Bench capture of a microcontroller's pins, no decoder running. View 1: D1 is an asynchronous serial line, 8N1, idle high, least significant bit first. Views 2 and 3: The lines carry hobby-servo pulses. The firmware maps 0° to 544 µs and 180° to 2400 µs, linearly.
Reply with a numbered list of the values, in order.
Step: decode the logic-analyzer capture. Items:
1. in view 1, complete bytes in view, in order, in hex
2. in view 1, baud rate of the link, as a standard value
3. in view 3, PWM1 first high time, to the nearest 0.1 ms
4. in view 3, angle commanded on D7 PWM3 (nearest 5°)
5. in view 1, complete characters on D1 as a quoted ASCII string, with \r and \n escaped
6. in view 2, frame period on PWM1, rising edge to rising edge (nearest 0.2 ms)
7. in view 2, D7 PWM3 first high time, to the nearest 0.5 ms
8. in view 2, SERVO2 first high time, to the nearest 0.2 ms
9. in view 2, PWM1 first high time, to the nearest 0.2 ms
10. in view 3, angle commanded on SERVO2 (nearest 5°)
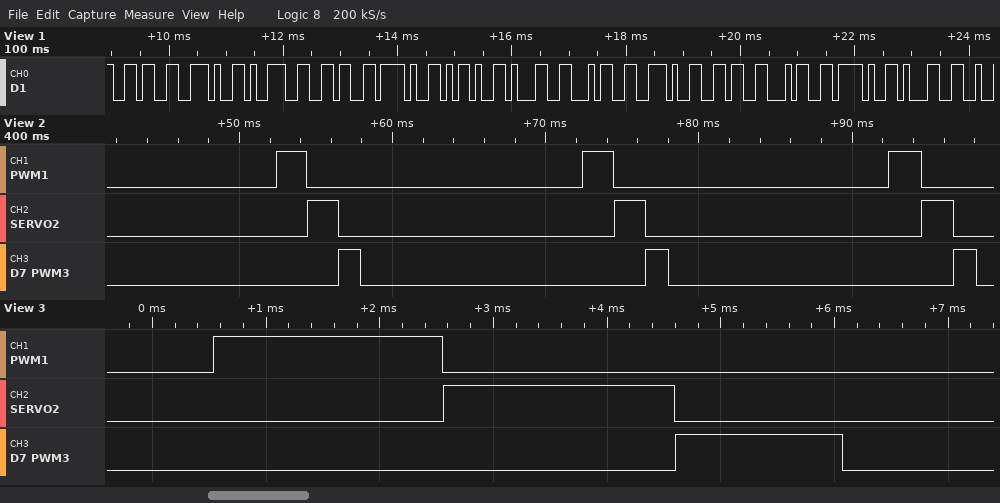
1. 36 2E 39 36 2F 2D 31 34 2E 36 34 2F 31
2. 9600 baud
3. 2.0 ms
4. 90°
5. "6.96/-14.64/1"
6. 20.0 ms
7. 1.5 ms
8. 2.0 ms
9. 2.0 ms
10. 145°
